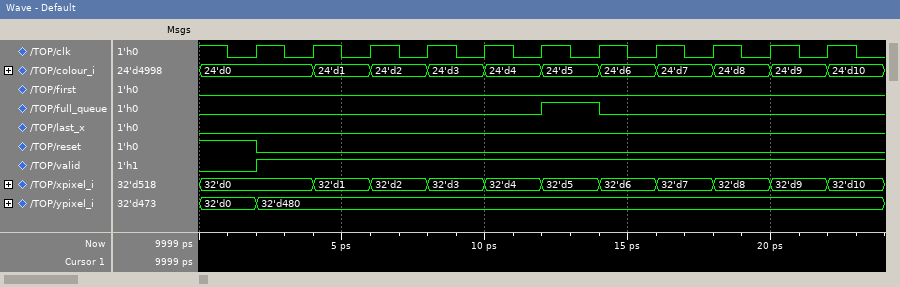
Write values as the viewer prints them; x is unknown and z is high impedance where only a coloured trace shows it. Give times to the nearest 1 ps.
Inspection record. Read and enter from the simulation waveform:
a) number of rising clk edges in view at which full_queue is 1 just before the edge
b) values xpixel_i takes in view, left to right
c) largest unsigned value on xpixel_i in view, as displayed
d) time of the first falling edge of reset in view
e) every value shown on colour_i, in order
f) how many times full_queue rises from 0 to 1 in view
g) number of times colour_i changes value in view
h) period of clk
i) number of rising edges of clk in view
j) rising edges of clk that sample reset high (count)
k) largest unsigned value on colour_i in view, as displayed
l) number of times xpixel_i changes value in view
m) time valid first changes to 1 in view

1
32'd0, 32'd1, 32'd2, 32'd3, 32'd4, 32'd5, 32'd6, 32'd7, 32'd8, 32'd9, 32'd10
32'd10
2 ps
24'd0, 24'd1, 24'd2, 24'd3, 24'd4, 24'd5, 24'd6, 24'd7, 24'd8, 24'd9, 24'd10
1
10
2 ps
11
1
24'd10
10
2 ps
